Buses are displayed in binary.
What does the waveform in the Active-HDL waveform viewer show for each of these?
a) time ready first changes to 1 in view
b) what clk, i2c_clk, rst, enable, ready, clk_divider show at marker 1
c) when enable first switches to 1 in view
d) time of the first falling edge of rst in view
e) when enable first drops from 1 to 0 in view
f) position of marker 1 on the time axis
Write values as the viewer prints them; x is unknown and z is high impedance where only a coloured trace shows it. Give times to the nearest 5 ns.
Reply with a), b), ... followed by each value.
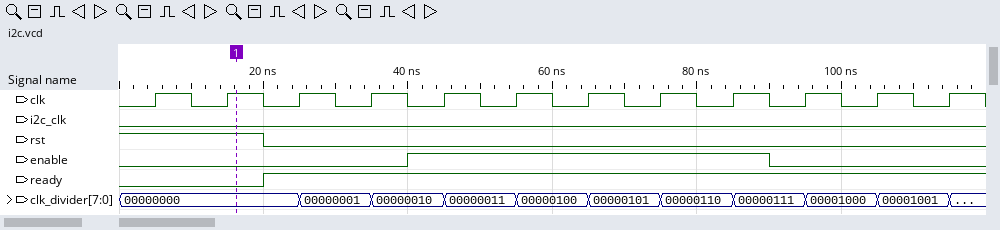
a) 20 ns
b) clk=1, i2c_clk=0, rst=1, enable=0, ready=0, clk_divider=00000000
c) 40 ns
d) 20 ns
e) 90 ns
f) 15 ns
